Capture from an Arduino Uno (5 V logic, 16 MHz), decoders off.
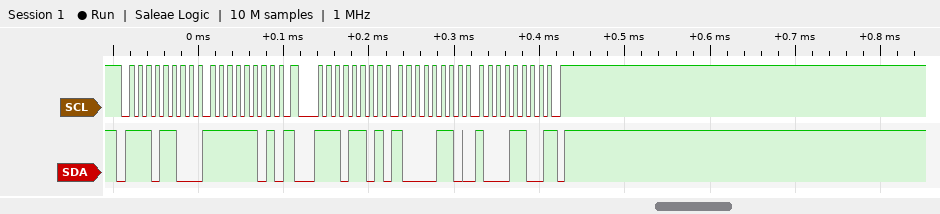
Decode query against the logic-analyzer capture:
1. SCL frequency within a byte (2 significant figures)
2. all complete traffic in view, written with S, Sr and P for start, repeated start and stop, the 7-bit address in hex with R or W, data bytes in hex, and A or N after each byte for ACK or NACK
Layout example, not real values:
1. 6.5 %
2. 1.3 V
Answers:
1. 100 kHz
2. S 76W A FD A Sr 76R A 86 A 8C N P
